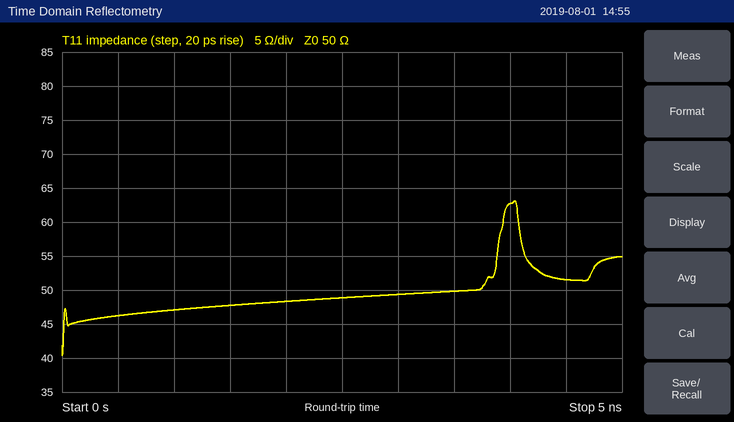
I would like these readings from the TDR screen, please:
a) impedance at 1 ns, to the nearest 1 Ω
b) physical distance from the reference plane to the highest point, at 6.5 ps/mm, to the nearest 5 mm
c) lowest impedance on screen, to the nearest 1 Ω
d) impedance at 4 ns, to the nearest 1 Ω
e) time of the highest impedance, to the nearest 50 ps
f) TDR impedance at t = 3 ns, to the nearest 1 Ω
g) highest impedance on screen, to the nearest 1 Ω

47 Ω
310 mm
40 Ω
63 Ω
4.05 ns
49 Ω
63 Ω
